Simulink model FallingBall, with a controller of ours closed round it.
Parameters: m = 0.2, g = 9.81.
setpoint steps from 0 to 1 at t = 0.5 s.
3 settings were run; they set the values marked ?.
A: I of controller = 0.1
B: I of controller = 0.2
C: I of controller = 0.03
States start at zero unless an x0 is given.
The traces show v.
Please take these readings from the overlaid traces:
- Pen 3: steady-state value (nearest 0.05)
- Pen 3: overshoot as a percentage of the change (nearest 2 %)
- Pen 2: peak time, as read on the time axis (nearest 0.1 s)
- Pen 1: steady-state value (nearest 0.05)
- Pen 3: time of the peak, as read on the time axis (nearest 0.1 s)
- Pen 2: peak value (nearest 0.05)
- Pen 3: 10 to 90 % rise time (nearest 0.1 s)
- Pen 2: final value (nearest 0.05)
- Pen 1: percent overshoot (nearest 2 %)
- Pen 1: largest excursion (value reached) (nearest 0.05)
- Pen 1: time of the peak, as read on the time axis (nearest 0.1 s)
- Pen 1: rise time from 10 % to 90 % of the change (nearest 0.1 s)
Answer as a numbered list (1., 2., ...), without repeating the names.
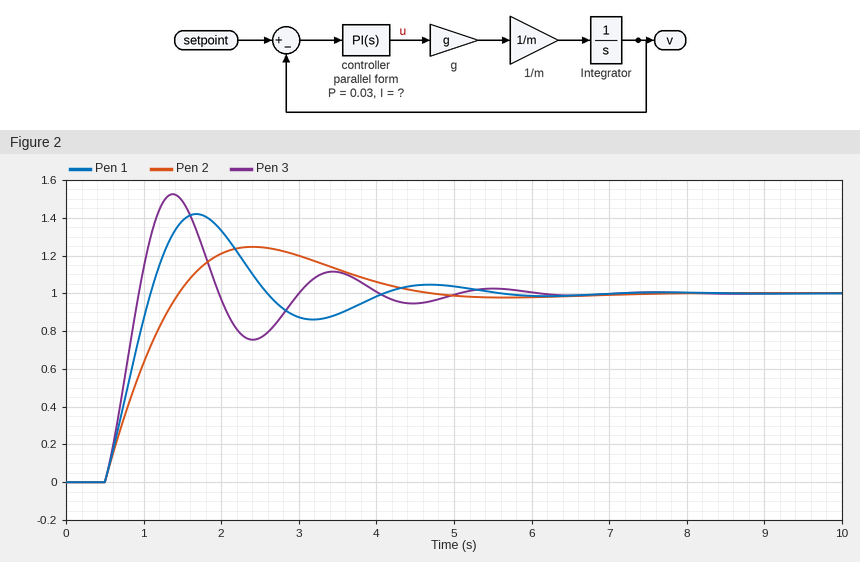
1. 1.00
2. 52 %
3. 2.4 s
4. 1.00
5. 1.4 s
6. 1.25
7. 0.3 s
8. 1.00
9. 42 %
10. 1.40
11. 1.7 s
12. 0.5 s
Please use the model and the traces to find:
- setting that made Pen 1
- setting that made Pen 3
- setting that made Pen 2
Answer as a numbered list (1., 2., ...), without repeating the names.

1. A
2. B
3. C
